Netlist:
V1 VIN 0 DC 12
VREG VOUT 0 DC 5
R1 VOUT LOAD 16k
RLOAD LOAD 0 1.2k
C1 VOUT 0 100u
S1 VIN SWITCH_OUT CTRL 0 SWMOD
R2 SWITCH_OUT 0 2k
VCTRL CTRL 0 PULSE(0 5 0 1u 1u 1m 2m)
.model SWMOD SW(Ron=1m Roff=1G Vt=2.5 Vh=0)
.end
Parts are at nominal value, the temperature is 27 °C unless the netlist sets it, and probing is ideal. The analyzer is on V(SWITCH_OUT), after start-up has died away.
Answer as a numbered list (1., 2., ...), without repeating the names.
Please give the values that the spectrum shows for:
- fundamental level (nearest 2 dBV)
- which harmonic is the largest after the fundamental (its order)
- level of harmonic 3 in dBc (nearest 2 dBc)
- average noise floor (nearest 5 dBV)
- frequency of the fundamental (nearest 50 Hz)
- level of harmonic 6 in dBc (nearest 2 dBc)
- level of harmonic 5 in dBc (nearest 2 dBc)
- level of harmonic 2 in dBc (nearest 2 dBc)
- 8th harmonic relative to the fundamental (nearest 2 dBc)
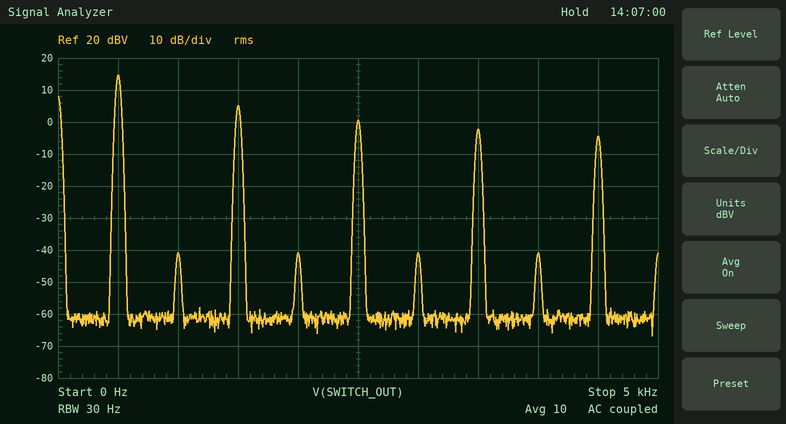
1. 14 dBV
2. 3
3. -10 dBc
4. -60 dBV
5. 500 Hz
6. -56 dBc
7. -14 dBc
8. -56 dBc
9. -56 dBc
